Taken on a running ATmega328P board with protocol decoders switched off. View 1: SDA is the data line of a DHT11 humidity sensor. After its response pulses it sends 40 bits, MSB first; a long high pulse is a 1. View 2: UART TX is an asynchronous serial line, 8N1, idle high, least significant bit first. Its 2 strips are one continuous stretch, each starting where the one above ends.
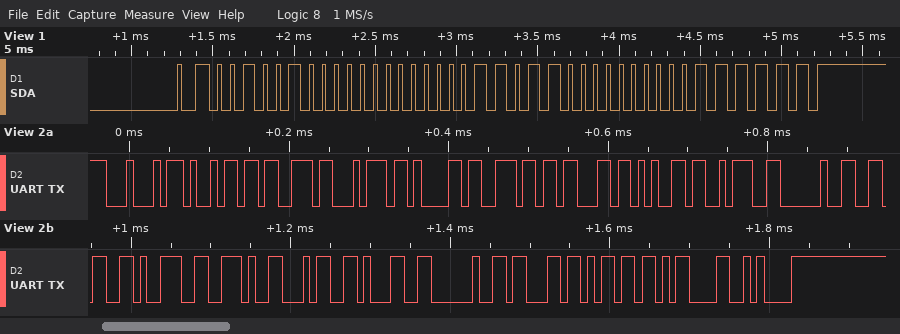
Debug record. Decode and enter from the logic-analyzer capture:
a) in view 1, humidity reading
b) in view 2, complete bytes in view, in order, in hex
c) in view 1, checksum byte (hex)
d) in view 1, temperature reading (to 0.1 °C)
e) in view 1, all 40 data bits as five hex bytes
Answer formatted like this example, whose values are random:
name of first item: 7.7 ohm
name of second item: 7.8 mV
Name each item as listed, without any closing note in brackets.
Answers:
in view 1, humidity reading: 36 %
in view 2, complete bytes in view, in order, in hex: 0x44 0x69 0x73 0x74 0x61 0x6E 0x63 0x65 0x3A 0x20 0x36 0x39 0x2E 0x34 0x31 0x20 0x63 0x6D 0x0D 0x0A
in view 1, checksum byte: 0x3F
in view 1, temperature reading: 27.0 °C
in view 1, all 40 data bits as five hex bytes: 24 00 1B 00 3F
